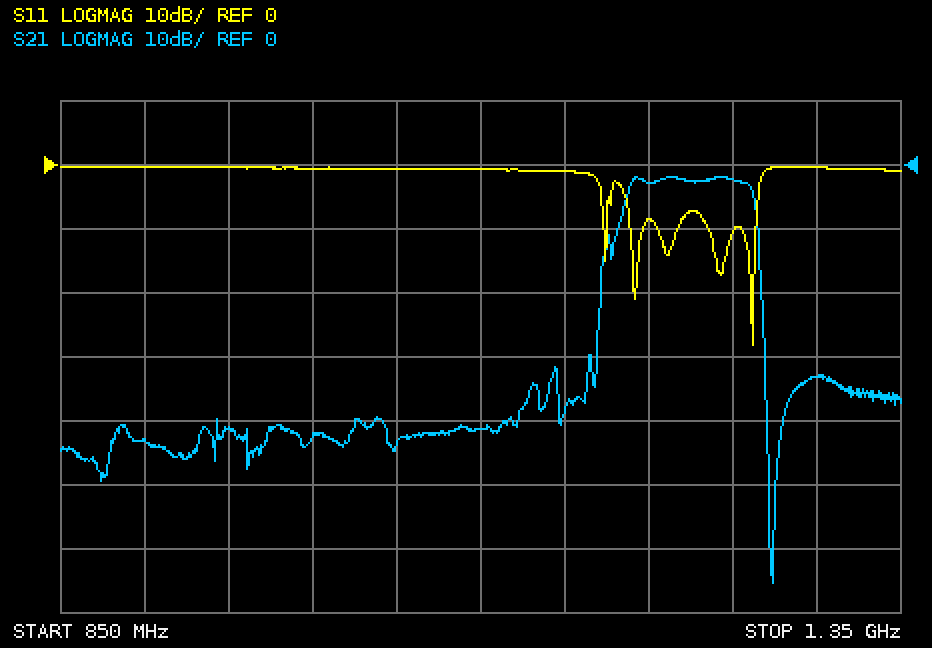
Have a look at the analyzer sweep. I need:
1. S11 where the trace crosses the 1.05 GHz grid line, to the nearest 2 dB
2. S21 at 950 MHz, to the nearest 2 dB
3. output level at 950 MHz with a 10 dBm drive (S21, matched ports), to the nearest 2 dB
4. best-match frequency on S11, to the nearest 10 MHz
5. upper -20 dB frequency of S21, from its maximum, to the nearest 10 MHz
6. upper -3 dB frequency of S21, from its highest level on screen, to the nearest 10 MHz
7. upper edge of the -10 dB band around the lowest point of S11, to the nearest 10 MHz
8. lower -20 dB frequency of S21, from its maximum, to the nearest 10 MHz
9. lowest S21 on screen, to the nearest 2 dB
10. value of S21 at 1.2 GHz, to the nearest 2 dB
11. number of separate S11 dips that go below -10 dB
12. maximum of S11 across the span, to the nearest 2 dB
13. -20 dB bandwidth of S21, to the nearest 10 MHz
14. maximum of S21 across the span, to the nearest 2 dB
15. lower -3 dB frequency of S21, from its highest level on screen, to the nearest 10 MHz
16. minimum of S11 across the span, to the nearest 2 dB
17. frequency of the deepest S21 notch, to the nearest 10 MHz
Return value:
0 dB
-42 dB
-32 dBm
1.26 GHz
1.27 GHz
1.26 GHz
1.26 GHz
1.17 GHz
-66 dB
-2 dB
5
0 dB
100 MHz
-2 dB
1.19 GHz
-28 dB
1.27 GHz
